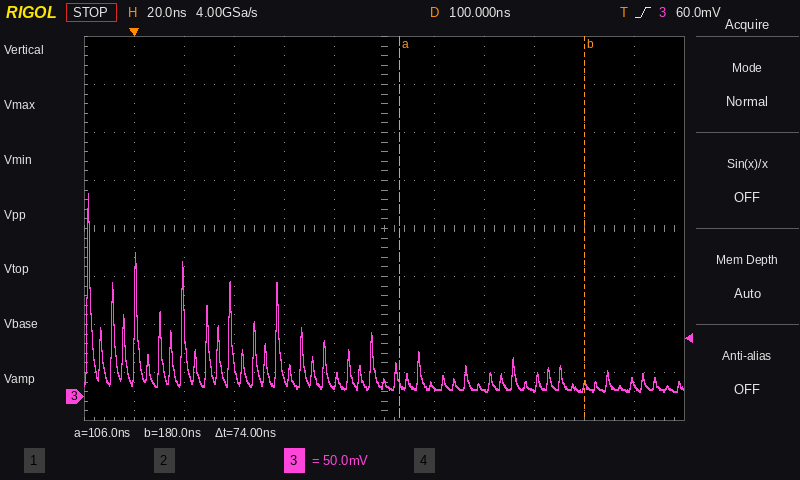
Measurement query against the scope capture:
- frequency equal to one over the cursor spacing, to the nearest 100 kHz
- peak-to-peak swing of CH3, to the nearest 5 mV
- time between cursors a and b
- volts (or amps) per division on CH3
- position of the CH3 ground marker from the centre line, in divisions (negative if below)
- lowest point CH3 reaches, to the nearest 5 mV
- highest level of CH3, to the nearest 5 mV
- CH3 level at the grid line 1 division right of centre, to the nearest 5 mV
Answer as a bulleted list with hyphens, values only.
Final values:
- 13.5 MHz
- 205 mV
- 74 ns
- 50 mV
- -3.5 div
- 5 mV
- 210 mV
- 10 mV
